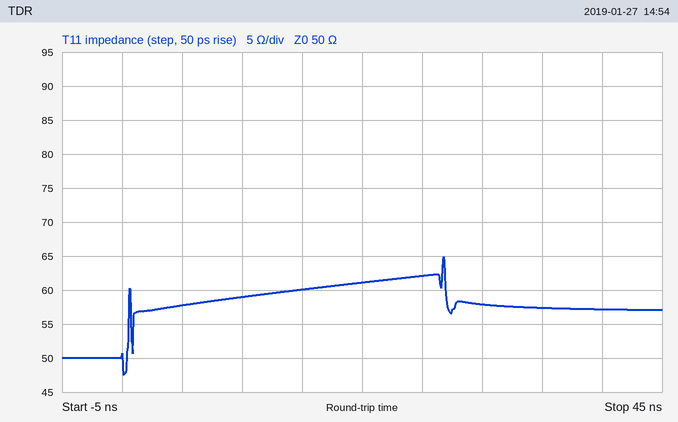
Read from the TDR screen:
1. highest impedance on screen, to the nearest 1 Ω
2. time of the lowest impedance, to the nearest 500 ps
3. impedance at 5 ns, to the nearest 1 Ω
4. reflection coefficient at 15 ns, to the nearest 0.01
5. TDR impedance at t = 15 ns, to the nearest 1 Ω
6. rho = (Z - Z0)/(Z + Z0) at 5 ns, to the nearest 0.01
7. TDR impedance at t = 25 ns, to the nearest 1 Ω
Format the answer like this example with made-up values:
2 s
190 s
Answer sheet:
65 Ω
0.0 ns
58 Ω
+0.09
60 Ω
+0.07
62 Ω
